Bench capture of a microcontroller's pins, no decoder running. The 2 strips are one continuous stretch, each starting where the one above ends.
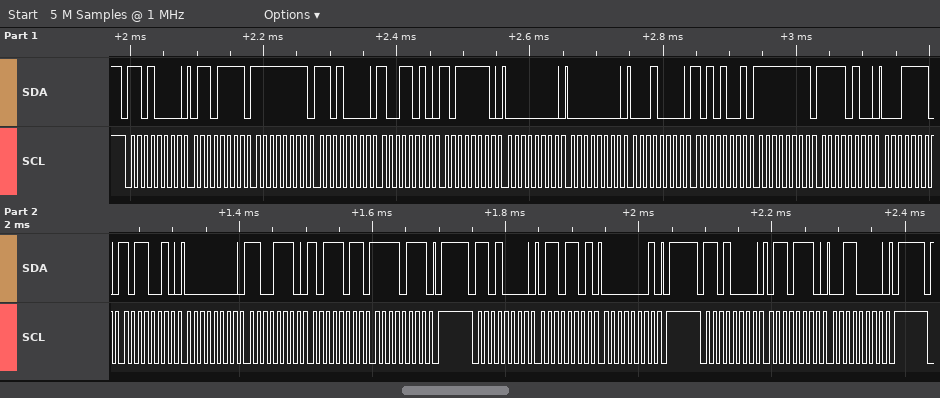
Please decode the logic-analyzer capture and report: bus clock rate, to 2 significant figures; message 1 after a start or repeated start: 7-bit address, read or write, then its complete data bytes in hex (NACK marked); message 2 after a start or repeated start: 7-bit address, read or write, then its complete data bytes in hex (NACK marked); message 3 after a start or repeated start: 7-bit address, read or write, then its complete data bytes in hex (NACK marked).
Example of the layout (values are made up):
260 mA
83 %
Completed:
100 kHz
0x68 write: 6F FF D0 9A BE 00 00 10 A9 FF F4 1E B2 00 CE BB F7
0x68 write: 6D 01
0x68 write: 6E 30
